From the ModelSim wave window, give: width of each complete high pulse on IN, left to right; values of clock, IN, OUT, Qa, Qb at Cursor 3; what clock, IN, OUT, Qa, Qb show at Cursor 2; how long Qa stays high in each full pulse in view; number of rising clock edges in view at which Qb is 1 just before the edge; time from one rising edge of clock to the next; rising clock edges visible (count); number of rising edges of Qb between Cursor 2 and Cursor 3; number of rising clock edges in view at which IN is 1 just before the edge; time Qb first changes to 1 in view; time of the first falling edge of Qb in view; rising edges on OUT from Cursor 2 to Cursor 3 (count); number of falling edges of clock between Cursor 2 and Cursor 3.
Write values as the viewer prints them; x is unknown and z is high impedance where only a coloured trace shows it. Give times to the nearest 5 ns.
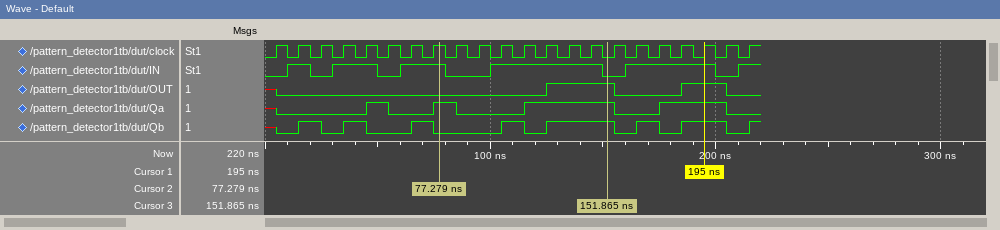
10 ns, 20 ns, 20 ns, 50 ns, 40 ns
clock=0, IN=0, OUT=1, Qa=1, Qb=1
clock=1, IN=1, OUT=0, Qa=1, Qb=0
10 ns, 10 ns, 40 ns, 30 ns
10
10 ns
22
2
15
15 ns
25 ns
1
8
